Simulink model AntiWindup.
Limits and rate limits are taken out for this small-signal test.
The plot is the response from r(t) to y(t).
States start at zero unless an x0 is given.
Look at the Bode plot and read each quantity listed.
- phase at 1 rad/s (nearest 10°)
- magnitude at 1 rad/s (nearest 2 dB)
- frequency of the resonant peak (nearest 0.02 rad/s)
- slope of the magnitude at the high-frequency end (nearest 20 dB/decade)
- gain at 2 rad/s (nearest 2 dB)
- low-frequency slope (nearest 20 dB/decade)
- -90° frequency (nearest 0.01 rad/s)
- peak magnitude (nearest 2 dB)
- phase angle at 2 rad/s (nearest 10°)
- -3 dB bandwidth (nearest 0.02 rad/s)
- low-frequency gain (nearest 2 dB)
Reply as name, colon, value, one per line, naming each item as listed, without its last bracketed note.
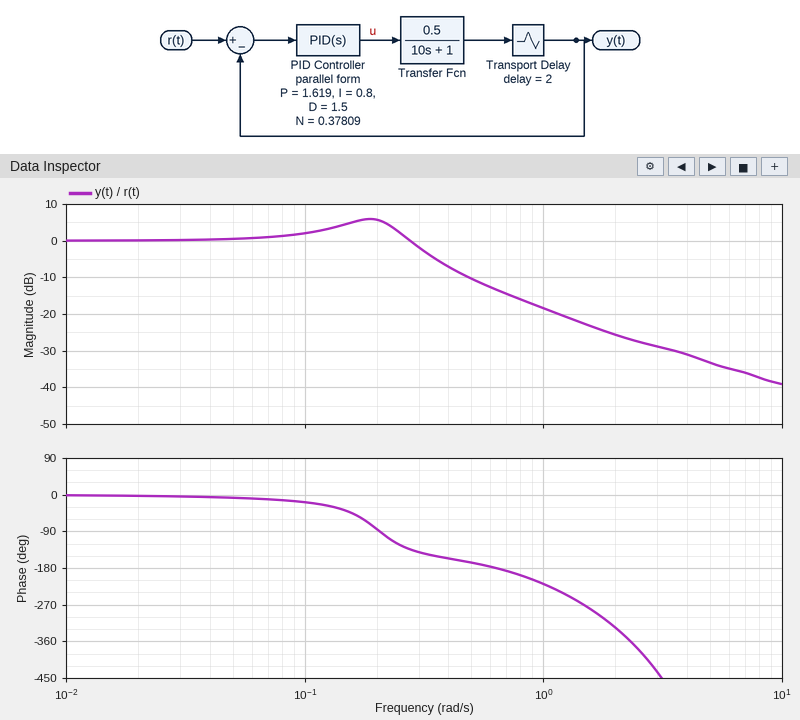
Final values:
phase at 1 rad/s: -220°
magnitude at 1 rad/s: -18 dB
frequency of the resonant peak: 0.18 rad/s
slope of the magnitude at the high-frequency end: -20 dB/decade
gain at 2 rad/s: -26 dB
low-frequency slope: 0 dB/decade
-90° frequency: 0.21 rad/s
peak magnitude: 6 dB
phase angle at 2 rad/s: -330°
-3 dB bandwidth: 0.32 rad/s
low-frequency gain: 0 dB
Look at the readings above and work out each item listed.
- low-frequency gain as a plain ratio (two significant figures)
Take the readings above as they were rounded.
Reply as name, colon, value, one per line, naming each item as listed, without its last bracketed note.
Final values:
low-frequency gain as a plain ratio: 1.0
